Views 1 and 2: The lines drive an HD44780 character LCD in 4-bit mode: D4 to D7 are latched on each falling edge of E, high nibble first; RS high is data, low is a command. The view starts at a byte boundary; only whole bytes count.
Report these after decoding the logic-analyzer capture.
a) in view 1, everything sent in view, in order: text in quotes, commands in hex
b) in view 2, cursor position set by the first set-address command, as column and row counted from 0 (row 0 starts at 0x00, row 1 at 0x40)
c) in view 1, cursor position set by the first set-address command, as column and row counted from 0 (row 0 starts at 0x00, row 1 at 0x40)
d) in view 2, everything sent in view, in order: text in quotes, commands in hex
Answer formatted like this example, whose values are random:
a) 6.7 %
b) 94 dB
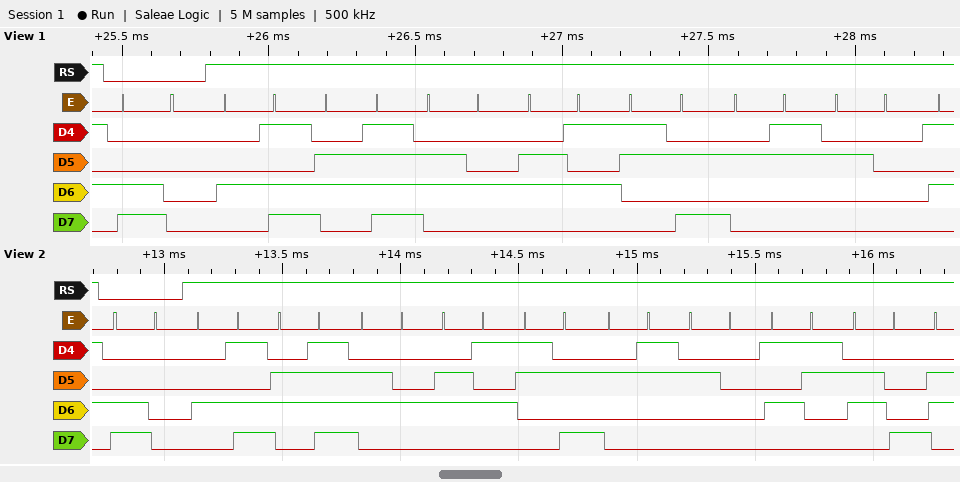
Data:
a) 0xC0 "Mode:# "
b) column 0, row 1
c) column 0, row 1
d) 0xC0 "Mode:# Sh"
